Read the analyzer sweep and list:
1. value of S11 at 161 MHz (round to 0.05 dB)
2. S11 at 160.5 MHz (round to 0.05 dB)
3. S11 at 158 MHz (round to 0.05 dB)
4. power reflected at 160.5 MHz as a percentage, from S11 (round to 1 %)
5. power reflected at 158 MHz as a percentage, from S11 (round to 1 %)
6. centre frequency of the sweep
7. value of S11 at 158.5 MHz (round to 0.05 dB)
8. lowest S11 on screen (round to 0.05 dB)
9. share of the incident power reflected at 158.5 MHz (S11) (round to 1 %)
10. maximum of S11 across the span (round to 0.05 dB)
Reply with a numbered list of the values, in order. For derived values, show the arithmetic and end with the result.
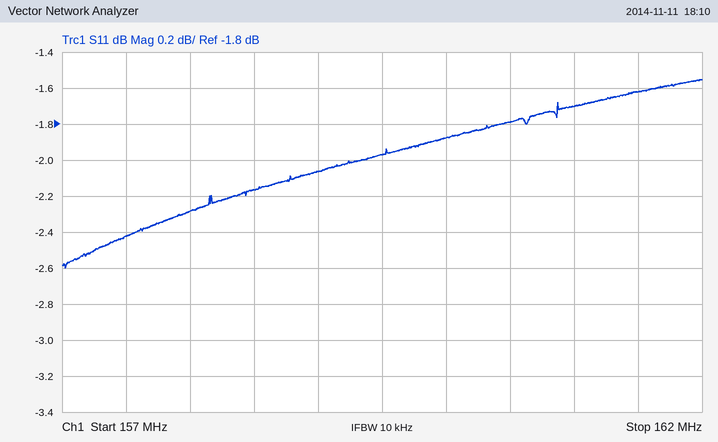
1. -1.70 dB
2. -1.80 dB
3. -2.30 dB
4. 10^(-1.8/10) ≈ 66 %
5. 10^(-2.3/10) ≈ 59 %
6. 159.5 MHz
7. -2.15 dB
8. -2.60 dB
9. 10^(-2.15/10) ≈ 61 %
10. -1.55 dB
